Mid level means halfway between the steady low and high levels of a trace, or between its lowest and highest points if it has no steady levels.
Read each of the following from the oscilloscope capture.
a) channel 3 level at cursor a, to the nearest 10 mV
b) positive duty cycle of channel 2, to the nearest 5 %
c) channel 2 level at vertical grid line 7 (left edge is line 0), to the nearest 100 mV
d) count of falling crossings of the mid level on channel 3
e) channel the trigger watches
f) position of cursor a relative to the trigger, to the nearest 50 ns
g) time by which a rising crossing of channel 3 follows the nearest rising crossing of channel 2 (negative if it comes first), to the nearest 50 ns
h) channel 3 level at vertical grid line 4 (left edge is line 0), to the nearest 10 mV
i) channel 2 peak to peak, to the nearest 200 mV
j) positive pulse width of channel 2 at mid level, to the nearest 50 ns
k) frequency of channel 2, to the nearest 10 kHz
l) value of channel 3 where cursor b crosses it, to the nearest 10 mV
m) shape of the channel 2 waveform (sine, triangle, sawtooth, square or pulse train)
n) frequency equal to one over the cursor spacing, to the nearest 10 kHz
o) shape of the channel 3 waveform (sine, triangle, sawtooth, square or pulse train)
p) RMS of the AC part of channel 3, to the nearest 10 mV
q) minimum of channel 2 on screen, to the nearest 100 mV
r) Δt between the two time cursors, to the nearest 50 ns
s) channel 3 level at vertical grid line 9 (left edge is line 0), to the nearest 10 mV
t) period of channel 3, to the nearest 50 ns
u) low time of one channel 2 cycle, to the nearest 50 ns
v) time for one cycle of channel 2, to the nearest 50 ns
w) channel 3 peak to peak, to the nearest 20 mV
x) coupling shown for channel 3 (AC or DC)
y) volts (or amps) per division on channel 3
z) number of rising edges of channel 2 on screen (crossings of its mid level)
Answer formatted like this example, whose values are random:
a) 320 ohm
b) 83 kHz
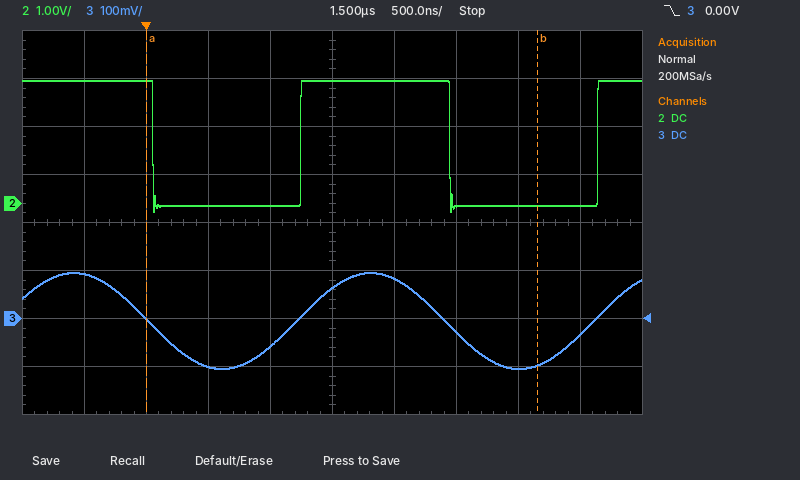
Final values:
a) 0 mV
b) 50 %
c) -100 mV
d) 2
e) channel 3
f) 0 ns
g) -50 ns
h) -60 mV
i) 2.8 V
j) 1.20 µs
k) 420 kHz
l) -100 mV
m) square
n) 320 kHz
o) sine
p) 70 mV
q) -200 mV
r) 3.15 µs
s) -30 mV
t) 2.40 µs
u) 1.20 µs
v) 2.40 µs
w) 200 mV
x) DC
y) 100 mV
z) 2
